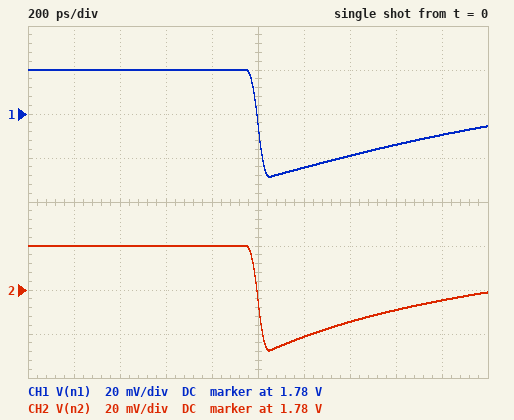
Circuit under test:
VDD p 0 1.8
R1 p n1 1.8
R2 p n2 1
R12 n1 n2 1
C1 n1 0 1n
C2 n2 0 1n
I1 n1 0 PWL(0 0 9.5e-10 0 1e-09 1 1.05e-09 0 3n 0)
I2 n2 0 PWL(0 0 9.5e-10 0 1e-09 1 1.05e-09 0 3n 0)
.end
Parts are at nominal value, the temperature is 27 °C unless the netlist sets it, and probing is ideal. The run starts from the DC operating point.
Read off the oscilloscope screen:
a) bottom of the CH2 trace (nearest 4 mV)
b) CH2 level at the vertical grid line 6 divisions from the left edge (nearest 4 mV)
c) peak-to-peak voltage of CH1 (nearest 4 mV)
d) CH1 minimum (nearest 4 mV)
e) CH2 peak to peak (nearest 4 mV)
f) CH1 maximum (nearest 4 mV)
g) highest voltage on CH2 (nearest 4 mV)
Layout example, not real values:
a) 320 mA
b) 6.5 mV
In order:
a) 1.752 V
b) 1.760 V
c) 48 mV
d) 1.752 V
e) 48 mV
f) 1.800 V
g) 1.800 V
